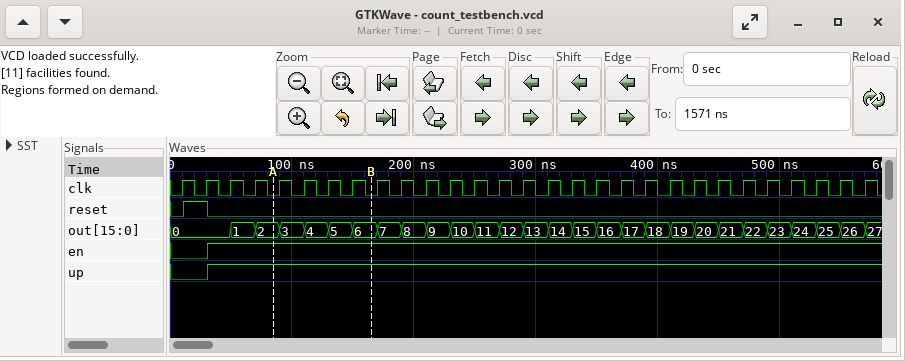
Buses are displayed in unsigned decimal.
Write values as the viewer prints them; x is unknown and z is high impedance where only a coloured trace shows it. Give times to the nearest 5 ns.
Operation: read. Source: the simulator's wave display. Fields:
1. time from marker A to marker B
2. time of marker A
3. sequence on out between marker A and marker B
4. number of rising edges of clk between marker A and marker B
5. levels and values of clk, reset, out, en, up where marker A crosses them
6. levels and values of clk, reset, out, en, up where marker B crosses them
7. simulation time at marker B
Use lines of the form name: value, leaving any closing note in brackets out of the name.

time from marker A to marker B: 80 ns
time of marker A: 85 ns
sequence on out between marker A and marker B: 2, 3, 4, 5, 6
number of rising edges of clk between marker A and marker B: 4
levels and values of clk, reset, out, en, up where marker A crosses them: clk=0, reset=0, out=2, en=1, up=1
levels and values of clk, reset, out, en, up where marker B crosses them: clk=0, reset=0, out=6, en=1, up=1
simulation time at marker B: 165 ns
